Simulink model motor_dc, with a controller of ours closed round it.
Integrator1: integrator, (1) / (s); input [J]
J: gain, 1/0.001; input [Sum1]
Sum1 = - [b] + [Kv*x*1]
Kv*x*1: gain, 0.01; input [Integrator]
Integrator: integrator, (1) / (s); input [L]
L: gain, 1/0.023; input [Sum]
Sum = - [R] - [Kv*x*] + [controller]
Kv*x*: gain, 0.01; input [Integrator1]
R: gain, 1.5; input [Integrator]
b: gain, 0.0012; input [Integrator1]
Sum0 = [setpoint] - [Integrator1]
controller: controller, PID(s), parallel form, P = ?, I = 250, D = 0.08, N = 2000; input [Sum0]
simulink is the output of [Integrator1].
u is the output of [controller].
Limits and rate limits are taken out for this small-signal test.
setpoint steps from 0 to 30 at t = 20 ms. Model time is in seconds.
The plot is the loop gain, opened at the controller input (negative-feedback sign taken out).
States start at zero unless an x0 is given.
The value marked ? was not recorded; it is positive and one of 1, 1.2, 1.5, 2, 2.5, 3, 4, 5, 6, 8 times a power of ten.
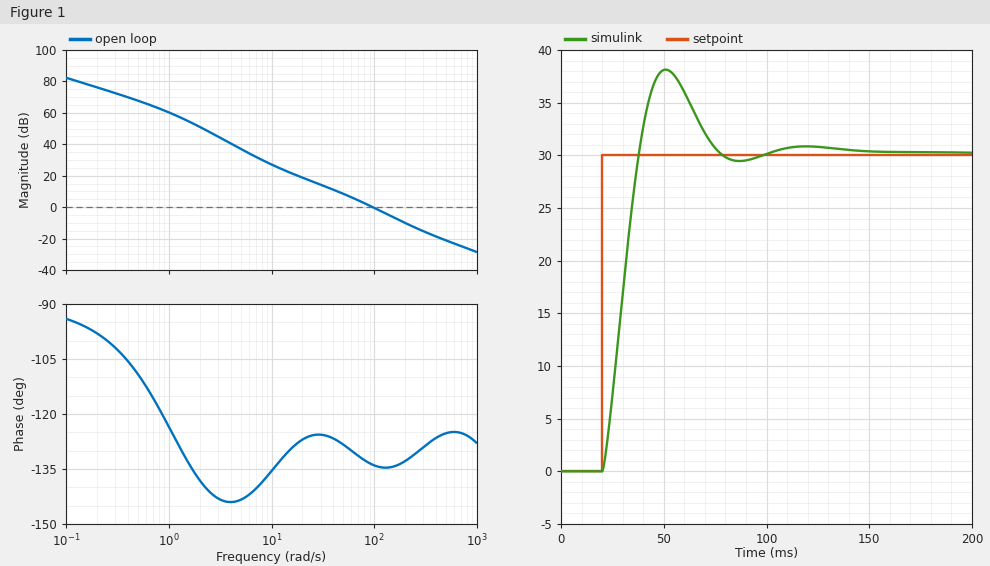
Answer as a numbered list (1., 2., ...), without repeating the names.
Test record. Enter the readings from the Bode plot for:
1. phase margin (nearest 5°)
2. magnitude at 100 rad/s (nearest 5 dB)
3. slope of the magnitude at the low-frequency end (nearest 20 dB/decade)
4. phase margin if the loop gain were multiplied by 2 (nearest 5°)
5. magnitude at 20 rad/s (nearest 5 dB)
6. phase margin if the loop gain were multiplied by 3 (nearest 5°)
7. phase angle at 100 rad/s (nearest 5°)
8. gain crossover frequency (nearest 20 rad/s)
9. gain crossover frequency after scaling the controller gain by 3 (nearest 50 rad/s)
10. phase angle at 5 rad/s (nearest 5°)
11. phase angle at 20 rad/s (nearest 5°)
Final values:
1. 45°
2. 0 dB
3. -20 dB/decade
4. 45°
5. 20 dB
6. 45°
7. -135°
8. 100 rad/s
9. 200 rad/s
10. -145°
11. -125°
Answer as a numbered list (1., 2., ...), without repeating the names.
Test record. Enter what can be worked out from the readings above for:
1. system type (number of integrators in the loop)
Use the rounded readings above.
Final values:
1. 1
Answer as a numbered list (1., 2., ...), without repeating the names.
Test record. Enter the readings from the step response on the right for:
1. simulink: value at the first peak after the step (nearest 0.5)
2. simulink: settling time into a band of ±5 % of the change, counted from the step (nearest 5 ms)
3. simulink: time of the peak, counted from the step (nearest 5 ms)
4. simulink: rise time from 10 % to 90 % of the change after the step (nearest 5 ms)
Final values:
1. 38.0
2. 50 ms
3. 30 ms
4. 15 ms
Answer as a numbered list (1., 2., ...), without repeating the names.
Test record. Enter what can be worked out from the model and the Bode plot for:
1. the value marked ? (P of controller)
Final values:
1. 25
